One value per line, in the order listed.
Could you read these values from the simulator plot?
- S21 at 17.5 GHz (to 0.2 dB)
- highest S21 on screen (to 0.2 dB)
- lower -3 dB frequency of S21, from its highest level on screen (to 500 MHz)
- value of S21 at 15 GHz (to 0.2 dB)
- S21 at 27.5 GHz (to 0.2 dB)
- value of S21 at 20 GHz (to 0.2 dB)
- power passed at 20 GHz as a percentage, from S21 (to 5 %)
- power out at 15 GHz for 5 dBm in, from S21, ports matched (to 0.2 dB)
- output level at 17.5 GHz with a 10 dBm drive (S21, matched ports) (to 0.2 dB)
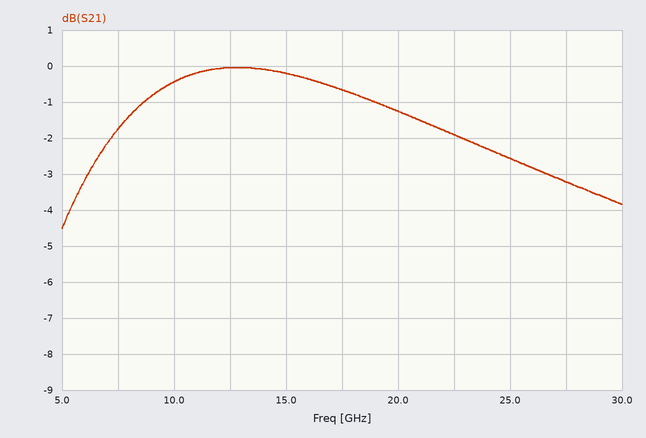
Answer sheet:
-0.6 dB
0.0 dB
6.0 GHz
-0.2 dB
-3.2 dB
-1.2 dB
75 %
4.8 dBm
9.4 dBm
